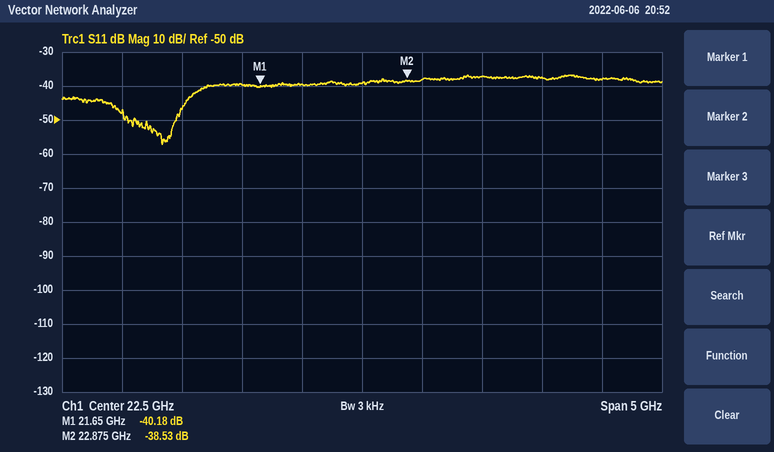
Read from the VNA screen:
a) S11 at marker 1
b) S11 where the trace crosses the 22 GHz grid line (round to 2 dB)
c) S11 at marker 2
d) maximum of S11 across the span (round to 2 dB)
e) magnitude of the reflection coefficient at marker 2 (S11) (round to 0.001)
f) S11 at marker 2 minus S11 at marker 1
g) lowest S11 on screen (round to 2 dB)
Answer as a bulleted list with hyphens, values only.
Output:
- -40.18 dB
- -40 dB
- -38.53 dB
- -36 dB
- 0.012
- 1.65 dB
- -58 dB
